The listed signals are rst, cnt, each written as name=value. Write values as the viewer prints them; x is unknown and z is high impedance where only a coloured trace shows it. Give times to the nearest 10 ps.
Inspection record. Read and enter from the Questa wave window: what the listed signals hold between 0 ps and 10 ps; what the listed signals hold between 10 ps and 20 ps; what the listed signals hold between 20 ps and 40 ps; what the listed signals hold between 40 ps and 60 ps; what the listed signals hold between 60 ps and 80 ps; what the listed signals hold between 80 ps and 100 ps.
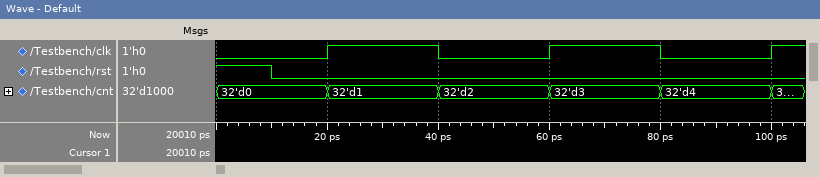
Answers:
rst=1, cnt=32'd0
rst=0, cnt=32'd0
rst=0, cnt=32'd1
rst=0, cnt=32'd2
rst=0, cnt=32'd3
rst=0, cnt=32'd4
